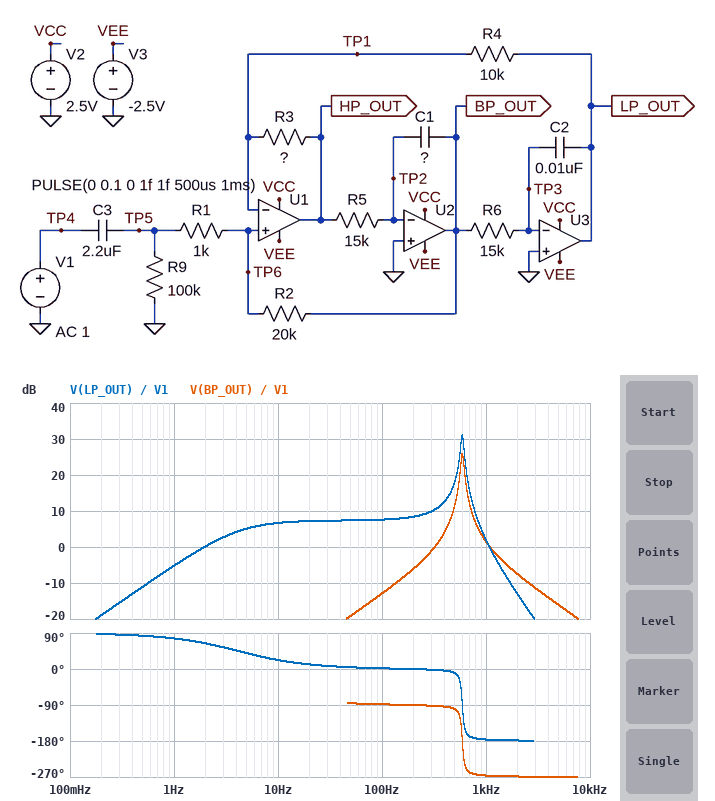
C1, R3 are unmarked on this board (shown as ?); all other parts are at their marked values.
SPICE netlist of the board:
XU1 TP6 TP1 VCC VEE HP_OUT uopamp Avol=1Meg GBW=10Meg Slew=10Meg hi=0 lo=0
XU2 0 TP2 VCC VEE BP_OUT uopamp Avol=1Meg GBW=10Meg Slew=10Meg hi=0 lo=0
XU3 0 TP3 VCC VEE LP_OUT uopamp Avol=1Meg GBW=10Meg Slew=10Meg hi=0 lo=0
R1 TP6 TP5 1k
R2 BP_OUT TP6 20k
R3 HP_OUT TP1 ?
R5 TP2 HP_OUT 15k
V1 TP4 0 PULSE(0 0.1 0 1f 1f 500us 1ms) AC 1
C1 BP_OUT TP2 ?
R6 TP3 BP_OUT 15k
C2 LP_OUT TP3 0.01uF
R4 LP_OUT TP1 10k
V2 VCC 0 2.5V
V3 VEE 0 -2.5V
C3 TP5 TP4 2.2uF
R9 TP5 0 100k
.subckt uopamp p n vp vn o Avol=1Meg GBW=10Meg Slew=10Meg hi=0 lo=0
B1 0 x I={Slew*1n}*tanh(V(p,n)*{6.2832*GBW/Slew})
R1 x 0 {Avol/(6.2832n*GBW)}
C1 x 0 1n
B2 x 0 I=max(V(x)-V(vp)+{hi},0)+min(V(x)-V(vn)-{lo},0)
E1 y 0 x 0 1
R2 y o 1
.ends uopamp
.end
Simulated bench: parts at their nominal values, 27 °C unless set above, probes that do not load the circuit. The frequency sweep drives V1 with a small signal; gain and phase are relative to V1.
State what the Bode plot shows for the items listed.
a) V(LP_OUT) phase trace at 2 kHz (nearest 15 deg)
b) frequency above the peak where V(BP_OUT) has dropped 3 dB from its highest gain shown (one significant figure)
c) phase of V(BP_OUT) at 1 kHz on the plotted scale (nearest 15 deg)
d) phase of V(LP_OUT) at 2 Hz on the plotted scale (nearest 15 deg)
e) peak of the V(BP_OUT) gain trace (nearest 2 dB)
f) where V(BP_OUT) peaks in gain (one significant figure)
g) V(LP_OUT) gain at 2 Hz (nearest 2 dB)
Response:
-180 deg
600 Hz
-270 deg
60 deg
26 dB
600 Hz
0 dB
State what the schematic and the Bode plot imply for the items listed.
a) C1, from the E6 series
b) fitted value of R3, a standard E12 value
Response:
22 nF
6.8 kΩ
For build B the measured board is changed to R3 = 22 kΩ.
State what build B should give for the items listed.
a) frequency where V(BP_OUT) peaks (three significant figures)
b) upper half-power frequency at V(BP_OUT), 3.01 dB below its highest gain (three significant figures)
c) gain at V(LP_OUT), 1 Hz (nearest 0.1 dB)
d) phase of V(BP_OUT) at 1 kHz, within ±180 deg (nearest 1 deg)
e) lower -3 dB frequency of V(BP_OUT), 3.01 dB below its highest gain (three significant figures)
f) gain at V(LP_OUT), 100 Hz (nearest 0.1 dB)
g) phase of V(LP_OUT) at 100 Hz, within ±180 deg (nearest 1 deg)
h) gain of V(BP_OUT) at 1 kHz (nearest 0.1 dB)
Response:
1.06 kHz
1.10 kHz
-9.8 dB
-119 deg
1.03 kHz
2.9 dB
2 deg
19.8 dB
